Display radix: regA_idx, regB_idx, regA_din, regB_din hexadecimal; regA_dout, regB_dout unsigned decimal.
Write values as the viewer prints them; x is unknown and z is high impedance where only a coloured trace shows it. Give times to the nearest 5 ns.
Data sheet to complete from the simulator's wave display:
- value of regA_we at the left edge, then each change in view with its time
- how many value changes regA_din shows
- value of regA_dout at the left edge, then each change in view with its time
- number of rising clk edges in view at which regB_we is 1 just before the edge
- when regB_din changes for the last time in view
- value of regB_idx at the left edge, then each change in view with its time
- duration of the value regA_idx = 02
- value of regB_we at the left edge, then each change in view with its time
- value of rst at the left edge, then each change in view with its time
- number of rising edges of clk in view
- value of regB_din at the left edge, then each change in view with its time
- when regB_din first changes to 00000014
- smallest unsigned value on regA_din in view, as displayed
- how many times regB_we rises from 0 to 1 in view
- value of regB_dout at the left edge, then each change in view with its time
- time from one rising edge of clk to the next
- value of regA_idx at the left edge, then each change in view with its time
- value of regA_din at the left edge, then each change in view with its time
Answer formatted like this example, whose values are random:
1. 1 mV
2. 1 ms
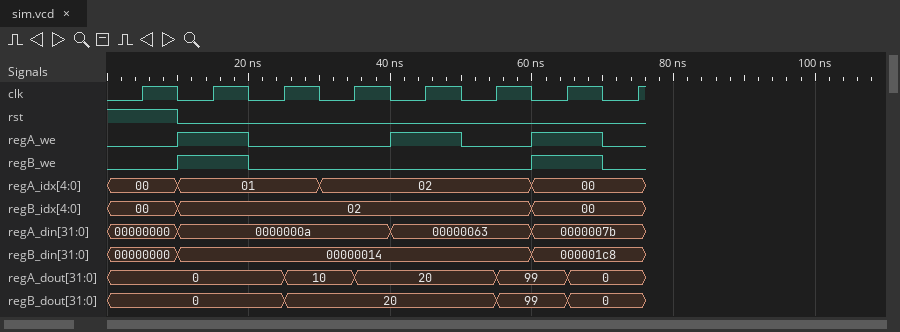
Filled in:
1. 0, 1 at 10 ns, 0 at 20 ns, 1 at 40 ns, 0 at 50 ns, 1 at 60 ns, 0 at 70 ns
2. 3
3. 0, 10 at 25 ns, 20 at 35 ns, 99 at 55 ns, 0 at 65 ns
4. 2
5. 60 ns
6. 00, 02 at 10 ns, 00 at 60 ns
7. 30 ns
8. 0, 1 at 10 ns, 0 at 20 ns, 1 at 60 ns, 0 at 70 ns
9. 1, 0 at 10 ns
10. 8
11. 00000000, 00000014 at 10 ns, 000001c8 at 60 ns
12. 10 ns
13. 00000000
14. 2
15. 0, 20 at 25 ns, 99 at 55 ns, 0 at 65 ns
16. 10 ns
17. 00, 01 at 10 ns, 02 at 30 ns, 00 at 60 ns
18. 00000000, 0000000a at 10 ns, 00000063 at 40 ns, 0000007b at 60 ns
